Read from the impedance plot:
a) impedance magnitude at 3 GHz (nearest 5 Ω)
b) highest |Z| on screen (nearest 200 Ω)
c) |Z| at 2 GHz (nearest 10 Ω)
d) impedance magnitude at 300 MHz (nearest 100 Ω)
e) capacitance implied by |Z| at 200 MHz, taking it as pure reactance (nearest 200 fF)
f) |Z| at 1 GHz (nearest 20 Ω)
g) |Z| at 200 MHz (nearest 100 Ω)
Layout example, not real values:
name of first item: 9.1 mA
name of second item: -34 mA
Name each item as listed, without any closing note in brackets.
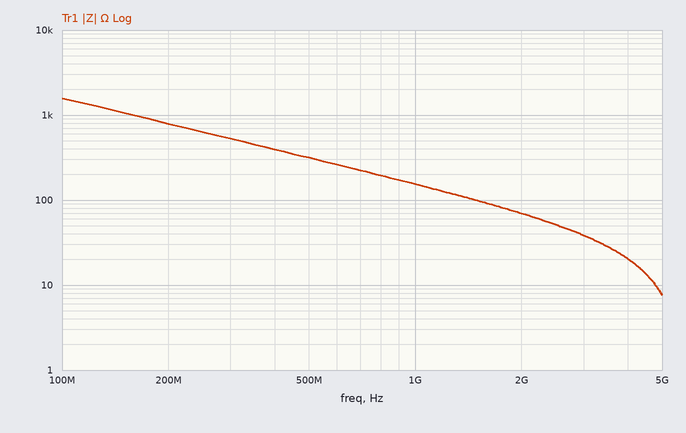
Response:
impedance magnitude at 3 GHz: 40 Ω
highest |Z| on screen: 1.6 kΩ
|Z| at 2 GHz: 70 Ω
impedance magnitude at 300 MHz: 500 Ω
capacitance implied by |Z| at 200 MHz, taking it as pure reactance: 1.0 pF
|Z| at 1 GHz: 160 Ω
|Z| at 200 MHz: 800 Ω
